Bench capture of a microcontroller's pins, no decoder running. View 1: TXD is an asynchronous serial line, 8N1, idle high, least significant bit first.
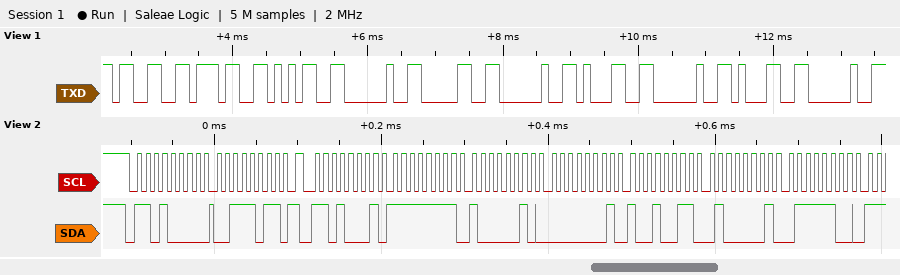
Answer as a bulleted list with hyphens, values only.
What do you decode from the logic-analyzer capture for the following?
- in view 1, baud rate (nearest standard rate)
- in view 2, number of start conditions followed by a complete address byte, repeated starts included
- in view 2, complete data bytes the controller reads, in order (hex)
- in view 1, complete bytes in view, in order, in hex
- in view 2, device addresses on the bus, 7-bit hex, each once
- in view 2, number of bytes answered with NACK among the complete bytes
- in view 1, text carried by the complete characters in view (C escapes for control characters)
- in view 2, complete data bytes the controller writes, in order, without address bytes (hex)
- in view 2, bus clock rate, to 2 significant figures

- 9600 baud
- 2
- FF 82 01 93 41 7C
- 0x33 0x37 0x35 0x20 0x30 0x20 0x31 0x20 0x31 0x20
- 0x68
- 0
- "375 0 1 1 "
- 3B
- 100 kHz
